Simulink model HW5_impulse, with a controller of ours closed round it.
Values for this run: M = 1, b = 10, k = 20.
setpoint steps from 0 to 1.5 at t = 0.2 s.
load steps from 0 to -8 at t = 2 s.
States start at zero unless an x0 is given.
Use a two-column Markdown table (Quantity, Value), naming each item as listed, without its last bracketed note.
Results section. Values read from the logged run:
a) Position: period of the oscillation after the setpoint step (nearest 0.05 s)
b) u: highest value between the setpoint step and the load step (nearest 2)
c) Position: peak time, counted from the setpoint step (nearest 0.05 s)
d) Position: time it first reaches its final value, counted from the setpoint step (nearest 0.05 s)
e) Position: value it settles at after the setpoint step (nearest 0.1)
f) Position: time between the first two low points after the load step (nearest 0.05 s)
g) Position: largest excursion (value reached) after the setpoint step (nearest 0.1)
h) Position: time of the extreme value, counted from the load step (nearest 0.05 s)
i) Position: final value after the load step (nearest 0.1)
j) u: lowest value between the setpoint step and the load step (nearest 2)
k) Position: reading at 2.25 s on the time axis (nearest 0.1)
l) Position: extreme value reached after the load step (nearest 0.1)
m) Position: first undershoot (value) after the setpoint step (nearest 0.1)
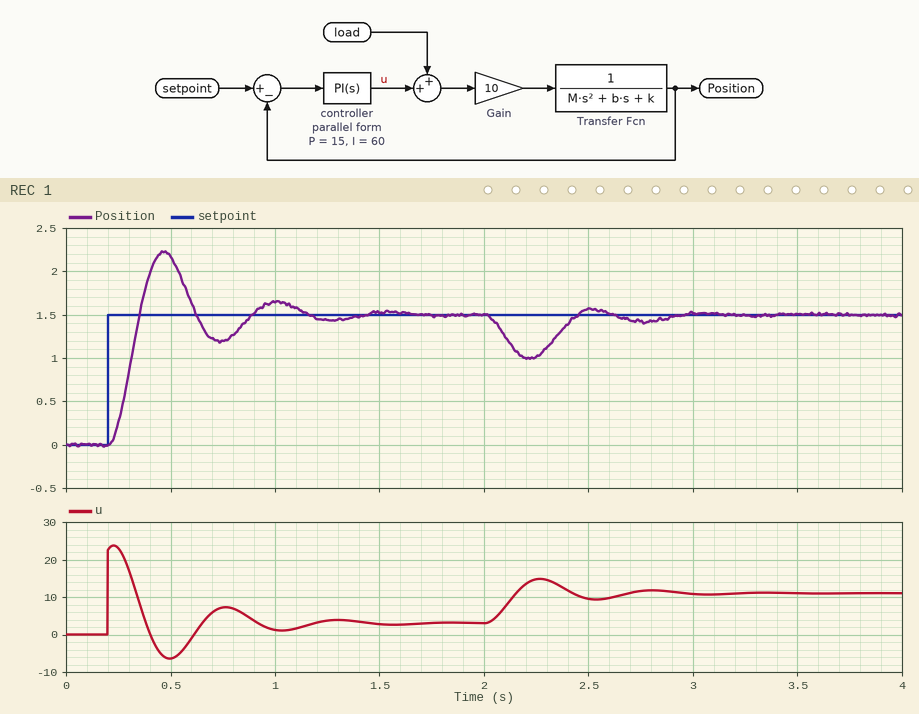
| Quantity | Value |
|---|---|
| Position: period of the oscillation after the setpoint step | 0.55 s |
| u: highest value between the setpoint step and the load step | 24 |
| Position: peak time, counted from the setpoint step | 0.25 s |
| Position: time it first reaches its final value, counted from the setpoint step | 0.15 s |
| Position: value it settles at after the setpoint step | 1.5 |
| Position: time between the first two low points after the load step | 0.55 s |
| Position: largest excursion (value reached) after the setpoint step | 2.2 |
| Position: time of the extreme value, counted from the load step | 0.20 s |
| Position: final value after the load step | 1.5 |
| u: lowest value between the setpoint step and the load step | -6 |
| Position: reading at 2.25 s on the time axis | 1.0 |
| Position: extreme value reached after the load step | 1.0 |
| Position: first undershoot (value) after the setpoint step | 1.2 |
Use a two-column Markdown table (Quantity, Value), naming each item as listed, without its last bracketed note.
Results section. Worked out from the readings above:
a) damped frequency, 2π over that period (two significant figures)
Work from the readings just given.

| Quantity | Value |
|---|---|
| damped frequency, 2π over that period | 11 rad/s |
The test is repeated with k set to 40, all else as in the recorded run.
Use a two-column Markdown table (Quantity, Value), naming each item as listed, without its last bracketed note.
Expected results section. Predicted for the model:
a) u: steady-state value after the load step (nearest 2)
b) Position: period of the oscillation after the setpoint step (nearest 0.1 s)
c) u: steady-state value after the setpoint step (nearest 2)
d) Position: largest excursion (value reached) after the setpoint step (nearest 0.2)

| Quantity | Value |
|---|---|
| u: steady-state value after the load step | 14 |
| Position: period of the oscillation after the setpoint step | 0.5 s |
| u: steady-state value after the setpoint step | 6 |
| Position: largest excursion (value reached) after the setpoint step | 2.0 |
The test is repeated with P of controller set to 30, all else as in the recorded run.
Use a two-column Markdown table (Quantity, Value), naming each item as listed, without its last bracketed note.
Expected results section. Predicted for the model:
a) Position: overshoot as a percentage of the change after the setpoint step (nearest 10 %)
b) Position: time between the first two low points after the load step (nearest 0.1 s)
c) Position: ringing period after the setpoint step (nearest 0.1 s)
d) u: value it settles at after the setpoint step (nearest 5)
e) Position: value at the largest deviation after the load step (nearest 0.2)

| Quantity | Value |
|---|---|
| Position: overshoot as a percentage of the change after the setpoint step | 50 % |
| Position: time between the first two low points after the load step | 0.4 s |
| Position: ringing period after the setpoint step | 0.4 s |
| u: value it settles at after the setpoint step | 5 |
| Position: value at the largest deviation after the load step | 1.2 |
